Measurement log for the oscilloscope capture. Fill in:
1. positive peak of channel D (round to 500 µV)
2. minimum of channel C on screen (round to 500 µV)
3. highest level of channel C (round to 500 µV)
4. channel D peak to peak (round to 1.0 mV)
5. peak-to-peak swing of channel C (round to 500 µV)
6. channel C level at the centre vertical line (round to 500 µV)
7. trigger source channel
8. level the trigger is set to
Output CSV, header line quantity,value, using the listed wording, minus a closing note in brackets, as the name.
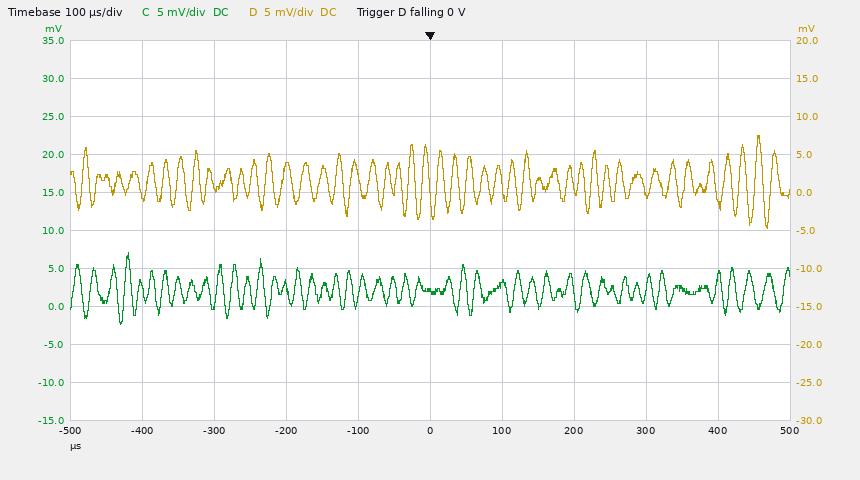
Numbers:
quantity,value
positive peak of channel D,7.5 mV
minimum of channel C on screen,-2.5 mV
highest level of channel C,7.0 mV
channel D peak to peak,12.0 mV
peak-to-peak swing of channel C,9.5 mV
channel C level at the centre vertical line,2.0 mV
trigger source channel,channel D
level the trigger is set to,0 V
